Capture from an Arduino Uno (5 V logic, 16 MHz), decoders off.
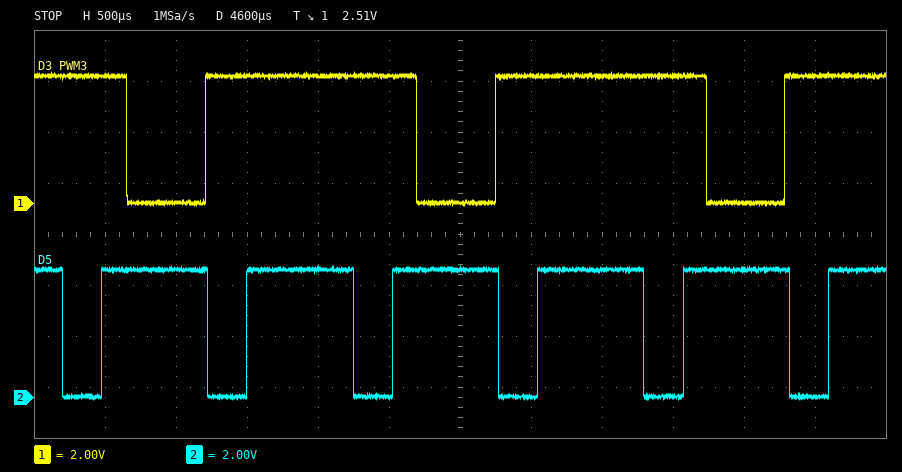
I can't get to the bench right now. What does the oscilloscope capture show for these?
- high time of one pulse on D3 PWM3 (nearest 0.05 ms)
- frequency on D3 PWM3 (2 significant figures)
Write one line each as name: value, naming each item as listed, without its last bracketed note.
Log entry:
high time of one pulse on D3 PWM3: 1.50 ms
frequency on D3 PWM3: 490 Hz
